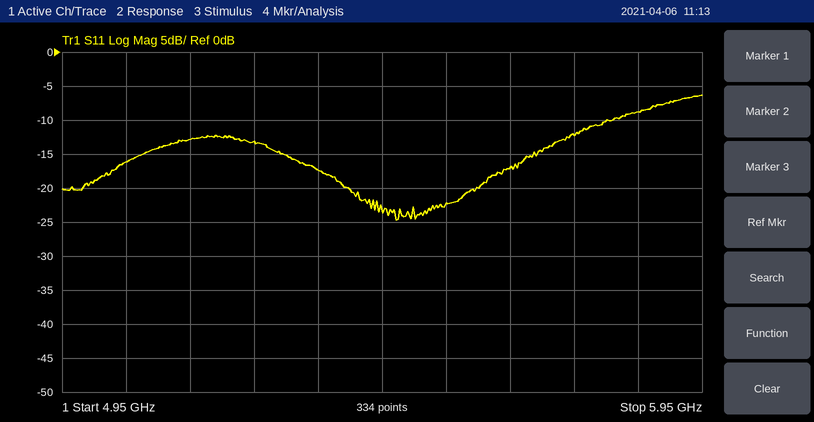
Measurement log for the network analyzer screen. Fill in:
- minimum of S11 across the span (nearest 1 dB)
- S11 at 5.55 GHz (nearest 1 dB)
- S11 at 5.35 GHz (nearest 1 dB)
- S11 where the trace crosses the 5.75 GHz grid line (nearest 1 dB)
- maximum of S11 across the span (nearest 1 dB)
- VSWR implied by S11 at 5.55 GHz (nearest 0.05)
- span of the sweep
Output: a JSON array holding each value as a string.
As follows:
["-25 dB", "-22 dB", "-17 dB", "-12 dB", "-6 dB", "1.15", "1 GHz"]
